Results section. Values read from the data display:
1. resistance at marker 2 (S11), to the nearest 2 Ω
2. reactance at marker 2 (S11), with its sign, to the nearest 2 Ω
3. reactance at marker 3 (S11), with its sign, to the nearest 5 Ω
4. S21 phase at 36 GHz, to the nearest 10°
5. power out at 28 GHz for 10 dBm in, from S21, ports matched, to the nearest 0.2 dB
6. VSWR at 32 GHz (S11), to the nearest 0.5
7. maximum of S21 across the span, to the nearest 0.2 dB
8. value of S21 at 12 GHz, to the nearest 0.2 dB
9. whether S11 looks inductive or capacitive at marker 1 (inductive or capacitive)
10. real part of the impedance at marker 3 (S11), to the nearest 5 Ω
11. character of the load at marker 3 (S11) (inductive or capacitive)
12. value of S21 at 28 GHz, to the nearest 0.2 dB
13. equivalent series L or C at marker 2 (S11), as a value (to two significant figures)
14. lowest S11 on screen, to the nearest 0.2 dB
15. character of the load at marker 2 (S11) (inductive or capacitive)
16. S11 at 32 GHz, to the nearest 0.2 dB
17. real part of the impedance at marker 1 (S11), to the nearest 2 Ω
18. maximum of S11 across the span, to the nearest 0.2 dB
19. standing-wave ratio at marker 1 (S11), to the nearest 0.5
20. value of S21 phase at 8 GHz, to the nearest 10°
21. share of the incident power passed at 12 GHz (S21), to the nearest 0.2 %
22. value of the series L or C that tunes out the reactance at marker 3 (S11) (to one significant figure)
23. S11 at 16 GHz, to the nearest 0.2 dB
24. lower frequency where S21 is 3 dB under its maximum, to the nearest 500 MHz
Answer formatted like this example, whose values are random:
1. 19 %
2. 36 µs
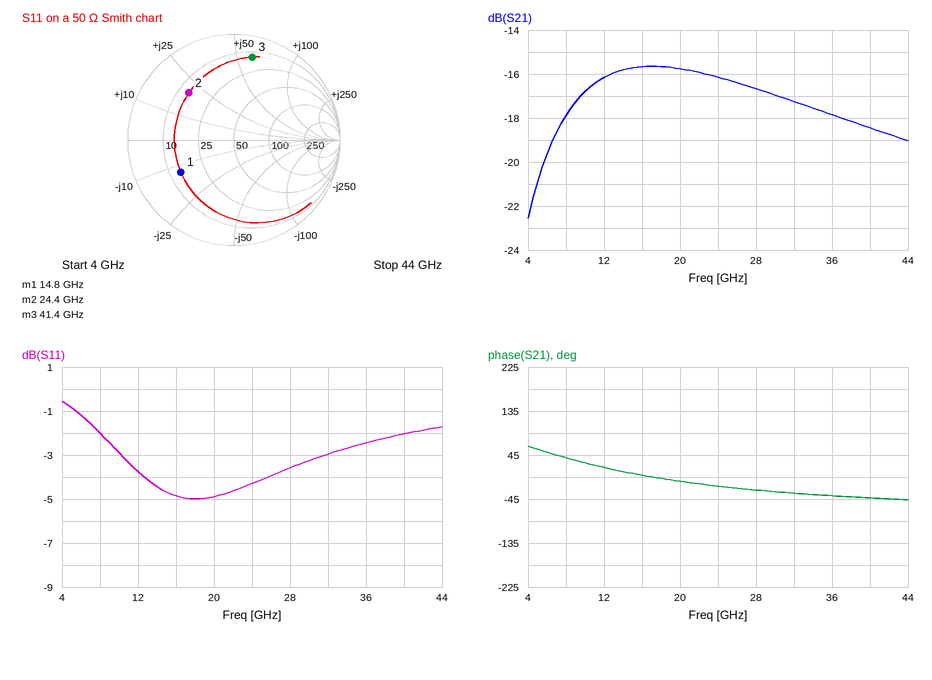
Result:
1. 14 Ω
2. +20 Ω
3. +60 Ω
4. -40°
5. -6.6 dBm
6. 6.0
7. -15.6 dB
8. -16.2 dB
9. capacitive
10. 15 Ω
11. inductive
12. -16.6 dB
13. 130 pH
14. -5.0 dB
15. inductive
16. -3.0 dB
17. 14 Ω
18. -0.6 dB
19. 4.0
20. 40°
21. 2.4 %
22. 60 fF
23. -4.8 dB
24. 7.0 GHz
